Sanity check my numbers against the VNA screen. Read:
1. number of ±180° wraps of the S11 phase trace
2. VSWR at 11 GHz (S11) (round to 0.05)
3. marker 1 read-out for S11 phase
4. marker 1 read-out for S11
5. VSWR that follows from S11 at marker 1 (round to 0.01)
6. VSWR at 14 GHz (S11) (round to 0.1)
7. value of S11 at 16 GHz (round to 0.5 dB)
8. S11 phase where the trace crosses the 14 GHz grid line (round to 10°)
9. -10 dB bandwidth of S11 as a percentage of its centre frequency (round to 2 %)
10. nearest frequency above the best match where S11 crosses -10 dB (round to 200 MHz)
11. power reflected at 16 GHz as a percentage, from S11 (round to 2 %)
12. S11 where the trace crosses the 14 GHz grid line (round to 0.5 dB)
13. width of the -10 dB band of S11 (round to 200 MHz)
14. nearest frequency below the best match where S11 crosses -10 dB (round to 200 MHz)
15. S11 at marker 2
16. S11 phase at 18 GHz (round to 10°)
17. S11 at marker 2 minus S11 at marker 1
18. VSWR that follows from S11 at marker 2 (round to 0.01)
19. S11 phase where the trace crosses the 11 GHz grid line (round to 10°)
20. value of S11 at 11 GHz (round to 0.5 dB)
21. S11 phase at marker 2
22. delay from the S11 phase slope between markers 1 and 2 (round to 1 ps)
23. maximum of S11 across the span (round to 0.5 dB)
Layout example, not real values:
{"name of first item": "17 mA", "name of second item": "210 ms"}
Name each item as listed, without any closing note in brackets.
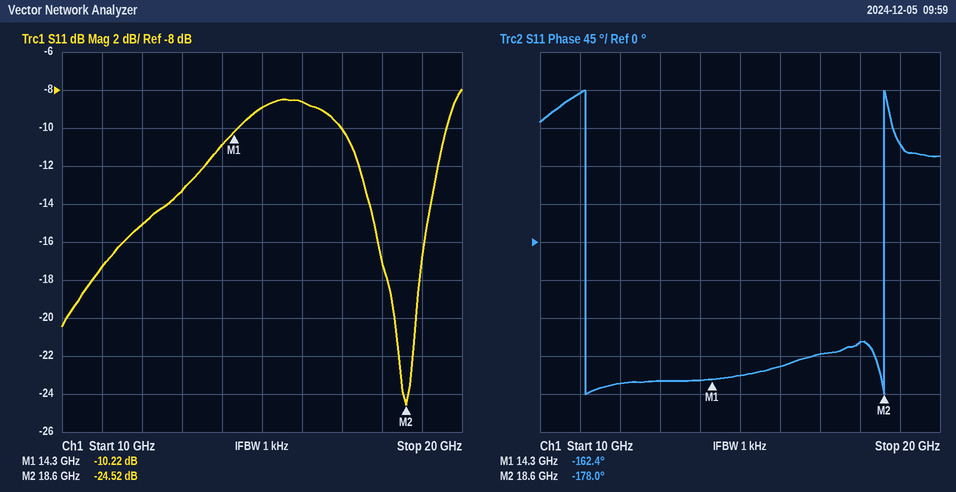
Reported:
{"number of ±180° wraps of the S11 phase trace": "2", "VSWR at 11 GHz (S11)": "1.30", "marker 1 read-out for S11 phase": "-162.4°", "marker 1 read-out for S11": "-10.22 dB", "VSWR that follows from S11 at marker 1": "1.89", "VSWR at 14 GHz (S11)": "1.8", "value of S11 at 16 GHz": "-8.5 dB", "S11 phase where the trace crosses the 14 GHz grid line": "-160°", "-10 dB bandwidth of S11 as a percentage of its centre frequency": "14 %", "nearest frequency above the best match where S11 crosses -10 dB": "19.6 GHz", "power reflected at 16 GHz as a percentage, from S11": "14 %", "S11 where the trace crosses the 14 GHz grid line": "-11.0 dB", "width of the -10 dB band of S11": "2.6 GHz", "nearest frequency below the best match where S11 crosses -10 dB": "17.0 GHz", "S11 at marker 2": "-24.52 dB", "S11 phase at 18 GHz": "-120°", "S11 at marker 2 minus S11 at marker 1": "-14.30 dB", "VSWR that follows from S11 at marker 2": "1.13", "S11 phase where the trace crosses the 11 GHz grid line": "180°", "value of S11 at 11 GHz": "-17.5 dB", "S11 phase at marker 2": "-178.0°", "delay from the S11 phase slope between markers 1 and 2": "10 ps", "maximum of S11 across the span": "-8.0 dB"}
